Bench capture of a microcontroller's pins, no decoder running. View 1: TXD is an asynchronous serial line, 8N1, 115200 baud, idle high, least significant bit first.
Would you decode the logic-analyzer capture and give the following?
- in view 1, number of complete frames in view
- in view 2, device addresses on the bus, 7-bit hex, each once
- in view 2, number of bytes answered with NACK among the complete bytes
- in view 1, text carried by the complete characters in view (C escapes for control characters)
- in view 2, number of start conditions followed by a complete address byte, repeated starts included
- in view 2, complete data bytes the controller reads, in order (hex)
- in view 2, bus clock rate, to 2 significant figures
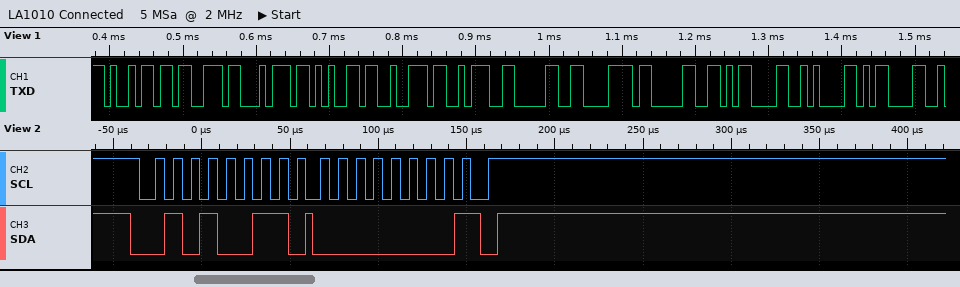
12
0x29
1
"ister:0x0\r\n\r"
1
00
100 kHz
